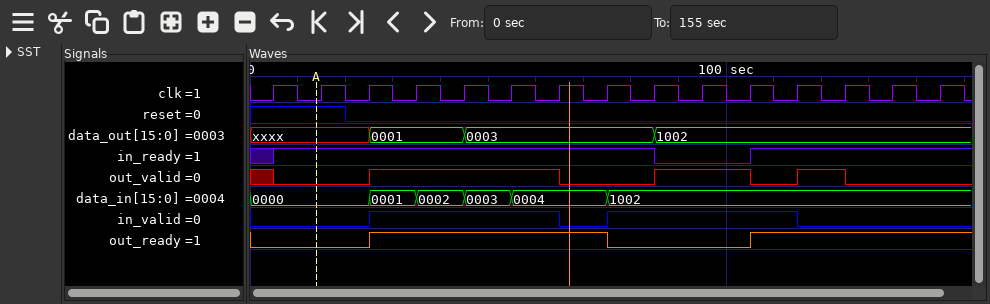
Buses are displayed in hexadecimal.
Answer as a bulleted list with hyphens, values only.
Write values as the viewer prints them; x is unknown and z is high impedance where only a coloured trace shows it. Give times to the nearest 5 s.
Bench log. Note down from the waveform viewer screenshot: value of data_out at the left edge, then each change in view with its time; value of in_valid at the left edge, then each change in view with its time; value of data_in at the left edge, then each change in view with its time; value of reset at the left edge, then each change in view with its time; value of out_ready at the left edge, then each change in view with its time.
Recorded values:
- xxxx, 0001 at 25 s, 0003 at 45 s, 1002 at 85 s
- 0, 1 at 25 s, 0 at 65 s, 1 at 75 s, 0 at 115 s
- 0000, 0001 at 25 s, 0002 at 35 s, 0003 at 45 s, 0004 at 55 s, 1002 at 75 s
- 1, 0 at 20 s
- 0, 1 at 25 s, 0 at 75 s, 1 at 105 s
